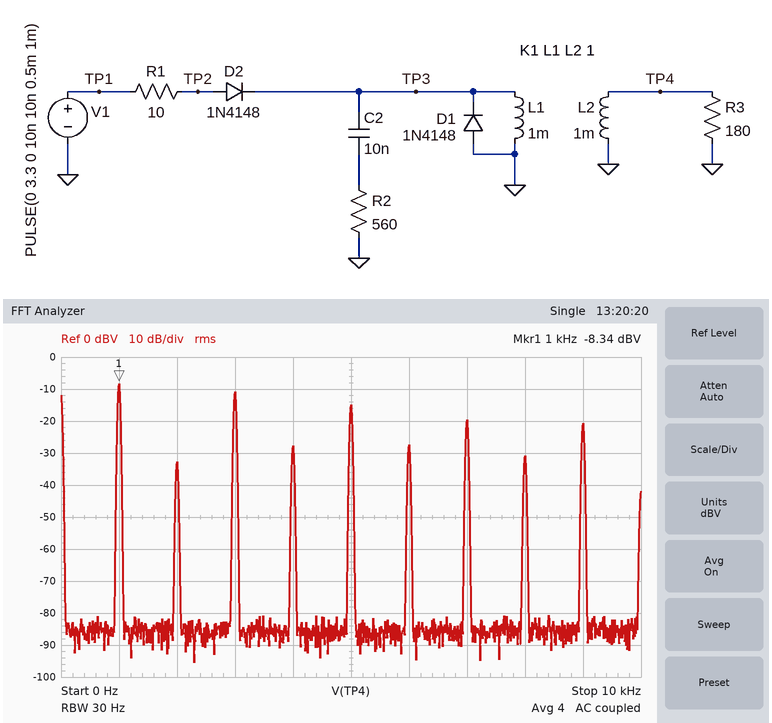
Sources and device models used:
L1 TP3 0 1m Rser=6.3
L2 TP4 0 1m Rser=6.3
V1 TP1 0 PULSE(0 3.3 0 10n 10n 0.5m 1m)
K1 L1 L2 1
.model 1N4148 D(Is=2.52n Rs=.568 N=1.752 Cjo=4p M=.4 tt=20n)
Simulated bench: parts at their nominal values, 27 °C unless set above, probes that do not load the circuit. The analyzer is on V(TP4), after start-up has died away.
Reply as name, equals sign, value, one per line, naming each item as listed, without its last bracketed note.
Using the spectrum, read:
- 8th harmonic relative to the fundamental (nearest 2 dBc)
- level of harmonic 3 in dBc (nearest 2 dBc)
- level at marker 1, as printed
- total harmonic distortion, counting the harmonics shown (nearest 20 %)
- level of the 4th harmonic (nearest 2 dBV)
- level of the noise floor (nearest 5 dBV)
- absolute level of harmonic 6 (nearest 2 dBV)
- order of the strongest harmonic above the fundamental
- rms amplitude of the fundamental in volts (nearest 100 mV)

8th harmonic relative to the fundamental = -22 dBc
level of harmonic 3 in dBc = -2 dBc
level at marker 1, as printed = -8.34 dBV
total harmonic distortion, counting the harmonics shown = 100 %
level of the 4th harmonic = -28 dBV
level of the noise floor = -85 dBV
absolute level of harmonic 6 = -28 dBV
order of the strongest harmonic above the fundamental = 3
rms amplitude of the fundamental in volts = 400 mV
